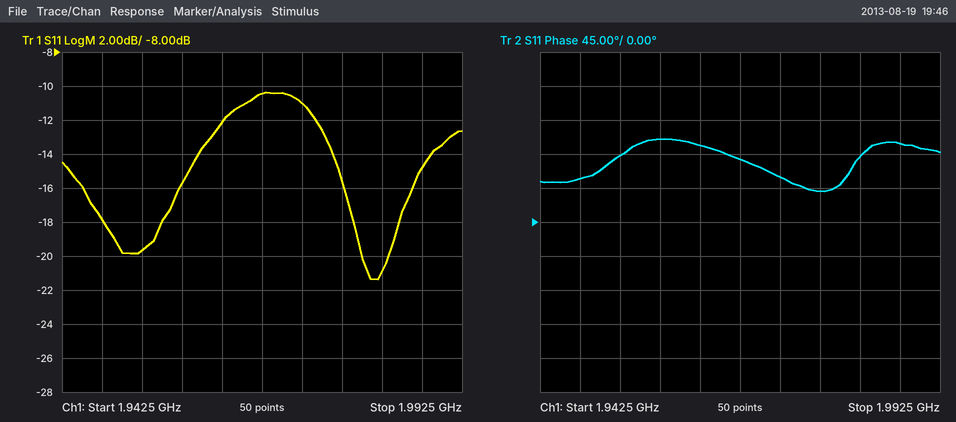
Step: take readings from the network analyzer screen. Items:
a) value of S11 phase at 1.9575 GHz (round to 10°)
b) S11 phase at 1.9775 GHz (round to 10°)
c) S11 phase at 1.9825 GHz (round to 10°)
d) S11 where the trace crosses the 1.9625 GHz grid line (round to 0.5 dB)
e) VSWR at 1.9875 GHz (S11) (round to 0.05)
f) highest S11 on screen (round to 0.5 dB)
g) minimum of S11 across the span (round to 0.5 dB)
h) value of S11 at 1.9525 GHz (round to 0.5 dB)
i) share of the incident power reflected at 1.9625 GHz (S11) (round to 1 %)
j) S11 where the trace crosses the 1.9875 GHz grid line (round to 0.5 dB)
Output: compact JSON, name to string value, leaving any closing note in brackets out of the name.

{"value of S11 phase at 1.9575 GHz": "110°", "S11 phase at 1.9775 GHz": "40°", "S11 phase at 1.9825 GHz": "90°", "S11 where the trace crosses the 1.9625 GHz grid line": "-12.0 dB", "VSWR at 1.9875 GHz (S11)": "1.45", "highest S11 on screen": "-10.5 dB", "minimum of S11 across the span": "-21.5 dB", "value of S11 at 1.9525 GHz": "-19.5 dB", "share of the incident power reflected at 1.9625 GHz (S11)": "6 %", "S11 where the trace crosses the 1.9875 GHz grid line": "-15.0 dB"}
